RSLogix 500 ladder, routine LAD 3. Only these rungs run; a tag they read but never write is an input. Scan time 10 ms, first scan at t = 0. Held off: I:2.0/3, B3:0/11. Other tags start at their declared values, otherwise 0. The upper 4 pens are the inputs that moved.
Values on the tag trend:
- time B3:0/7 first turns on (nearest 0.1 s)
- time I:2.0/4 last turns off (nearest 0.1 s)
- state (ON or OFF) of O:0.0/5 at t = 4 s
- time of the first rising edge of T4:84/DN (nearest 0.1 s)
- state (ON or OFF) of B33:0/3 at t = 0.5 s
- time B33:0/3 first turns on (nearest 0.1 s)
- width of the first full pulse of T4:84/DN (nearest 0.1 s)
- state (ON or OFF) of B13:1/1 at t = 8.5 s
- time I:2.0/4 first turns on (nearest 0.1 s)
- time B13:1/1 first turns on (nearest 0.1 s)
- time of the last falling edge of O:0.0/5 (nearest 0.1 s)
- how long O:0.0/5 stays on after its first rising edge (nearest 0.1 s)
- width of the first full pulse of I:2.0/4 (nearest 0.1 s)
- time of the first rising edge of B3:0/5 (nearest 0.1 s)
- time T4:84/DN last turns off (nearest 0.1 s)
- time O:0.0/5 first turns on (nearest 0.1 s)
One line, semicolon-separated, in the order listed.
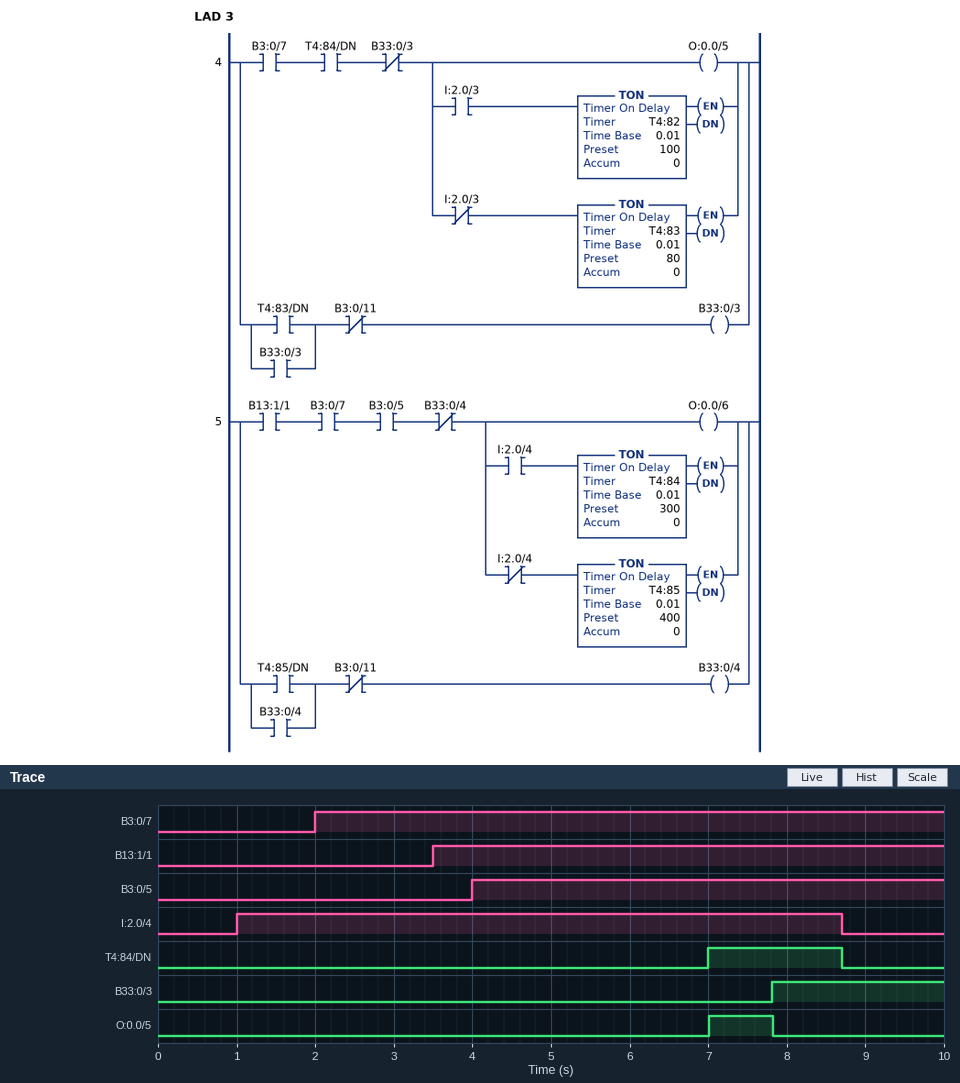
2.0 s; 8.7 s; OFF; 7.0 s; OFF; 7.8 s; 1.7 s; ON; 1.0 s; 3.5 s; 7.8 s; 0.8 s; 7.7 s; 4.0 s; 8.7 s; 7.0 s
